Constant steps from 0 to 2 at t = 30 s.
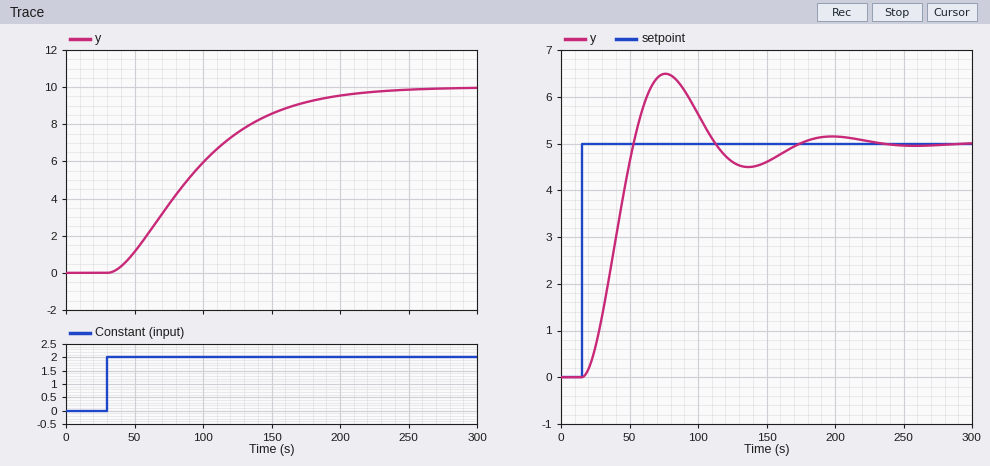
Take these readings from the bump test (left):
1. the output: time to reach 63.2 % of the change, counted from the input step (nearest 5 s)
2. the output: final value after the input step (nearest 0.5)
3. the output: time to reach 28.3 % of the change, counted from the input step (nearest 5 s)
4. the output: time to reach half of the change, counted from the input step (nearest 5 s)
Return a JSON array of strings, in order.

["75 s", "10.0", "35 s", "60 s"]
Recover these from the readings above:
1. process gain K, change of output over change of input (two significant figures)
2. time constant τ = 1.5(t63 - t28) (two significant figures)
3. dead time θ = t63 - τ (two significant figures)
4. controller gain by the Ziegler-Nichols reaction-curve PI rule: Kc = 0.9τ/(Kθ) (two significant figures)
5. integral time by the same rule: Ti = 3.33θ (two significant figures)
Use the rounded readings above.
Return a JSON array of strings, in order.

["5.0", "60 s", "15 s", "0.72", "50 s"]
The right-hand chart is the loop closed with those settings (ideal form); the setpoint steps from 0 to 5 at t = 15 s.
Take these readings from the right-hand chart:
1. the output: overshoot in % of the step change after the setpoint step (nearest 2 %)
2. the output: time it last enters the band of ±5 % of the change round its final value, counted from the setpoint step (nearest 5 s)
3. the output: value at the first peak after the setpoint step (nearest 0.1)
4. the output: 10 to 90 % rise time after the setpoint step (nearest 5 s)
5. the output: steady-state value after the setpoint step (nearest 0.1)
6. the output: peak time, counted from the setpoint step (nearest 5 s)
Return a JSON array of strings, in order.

["30 %", "145 s", "6.5", "25 s", "5.0", "60 s"]
